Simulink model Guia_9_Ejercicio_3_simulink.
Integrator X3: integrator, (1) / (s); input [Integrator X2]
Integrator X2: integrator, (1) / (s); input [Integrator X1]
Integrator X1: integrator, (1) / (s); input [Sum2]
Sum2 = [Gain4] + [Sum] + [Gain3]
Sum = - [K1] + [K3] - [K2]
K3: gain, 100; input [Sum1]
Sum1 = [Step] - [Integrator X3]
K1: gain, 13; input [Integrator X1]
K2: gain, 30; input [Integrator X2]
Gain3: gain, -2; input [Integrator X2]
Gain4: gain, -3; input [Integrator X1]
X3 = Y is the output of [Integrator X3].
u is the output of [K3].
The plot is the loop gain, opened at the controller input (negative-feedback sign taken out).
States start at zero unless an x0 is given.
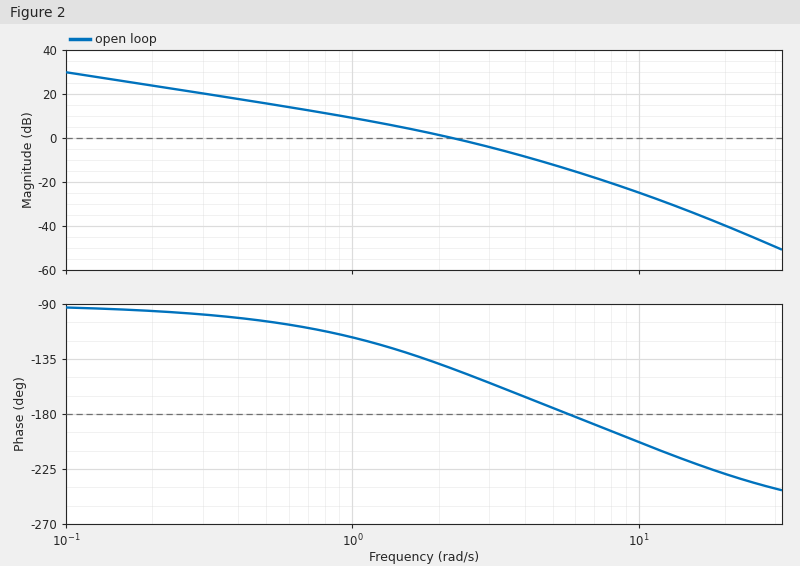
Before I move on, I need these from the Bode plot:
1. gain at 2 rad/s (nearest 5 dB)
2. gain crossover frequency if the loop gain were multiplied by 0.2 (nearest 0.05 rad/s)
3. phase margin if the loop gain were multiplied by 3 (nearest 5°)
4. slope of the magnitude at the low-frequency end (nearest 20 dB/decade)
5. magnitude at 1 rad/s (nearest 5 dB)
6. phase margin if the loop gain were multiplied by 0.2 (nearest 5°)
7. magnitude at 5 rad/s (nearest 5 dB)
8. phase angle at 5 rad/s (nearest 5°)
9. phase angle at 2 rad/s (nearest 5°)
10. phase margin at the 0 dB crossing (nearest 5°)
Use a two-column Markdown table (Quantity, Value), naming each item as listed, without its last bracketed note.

| Quantity | Value |
|---|---|
| gain at 2 rad/s | 0 dB |
| gain crossover frequency if the loop gain were multiplied by 0.2 | 0.60 rad/s |
| phase margin if the loop gain were multiplied by 3 | 10° |
| slope of the magnitude at the low-frequency end | -20 dB/decade |
| magnitude at 1 rad/s | 10 dB |
| phase margin if the loop gain were multiplied by 0.2 | 75° |
| magnitude at 5 rad/s | -10 dB |
| phase angle at 5 rad/s | -175° |
| phase angle at 2 rad/s | -140° |
| phase margin at the 0 dB crossing | 35° |
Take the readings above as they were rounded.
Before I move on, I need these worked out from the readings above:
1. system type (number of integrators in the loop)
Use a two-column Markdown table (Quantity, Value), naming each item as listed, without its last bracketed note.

| Quantity | Value |
|---|---|
| system type | 1 |
